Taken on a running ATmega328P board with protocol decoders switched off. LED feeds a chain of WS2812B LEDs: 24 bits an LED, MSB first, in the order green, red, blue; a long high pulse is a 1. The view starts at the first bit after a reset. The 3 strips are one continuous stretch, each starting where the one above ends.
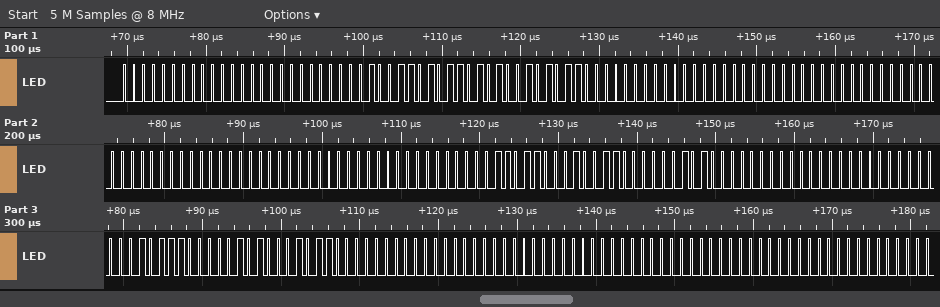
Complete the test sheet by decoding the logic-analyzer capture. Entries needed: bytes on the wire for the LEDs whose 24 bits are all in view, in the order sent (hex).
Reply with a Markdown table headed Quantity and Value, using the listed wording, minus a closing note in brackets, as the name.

| Quantity | Value |
|---|---|
| bytes on the wire for the LEDs whose 24 bits are all in view, in the order sent | 00 00 00 4D 6A 56 00 00 00 00 00 00 00 00 00 36 26 05 00 00 00 2E 0A 2C 00 00 00 00 00 00 |
